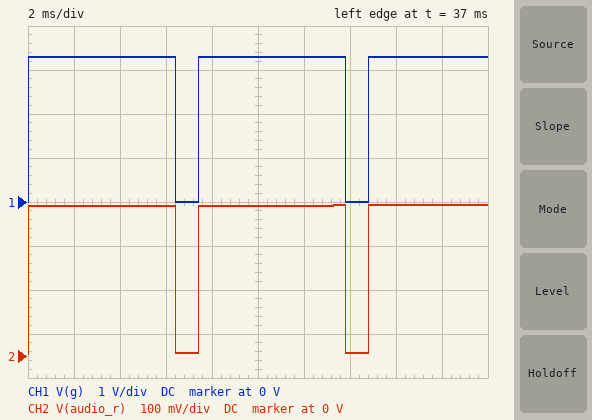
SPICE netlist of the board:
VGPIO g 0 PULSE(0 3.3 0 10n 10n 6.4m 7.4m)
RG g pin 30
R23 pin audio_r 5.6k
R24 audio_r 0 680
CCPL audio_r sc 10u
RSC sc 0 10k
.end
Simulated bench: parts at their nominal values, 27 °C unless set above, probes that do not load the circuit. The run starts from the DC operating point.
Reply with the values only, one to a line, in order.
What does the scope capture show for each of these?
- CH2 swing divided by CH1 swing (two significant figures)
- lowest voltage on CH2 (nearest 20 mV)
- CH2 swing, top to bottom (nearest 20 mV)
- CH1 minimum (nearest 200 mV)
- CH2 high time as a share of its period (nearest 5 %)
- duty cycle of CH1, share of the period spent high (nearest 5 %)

0.10
0 V
340 mV
0 V
85 %
85 %
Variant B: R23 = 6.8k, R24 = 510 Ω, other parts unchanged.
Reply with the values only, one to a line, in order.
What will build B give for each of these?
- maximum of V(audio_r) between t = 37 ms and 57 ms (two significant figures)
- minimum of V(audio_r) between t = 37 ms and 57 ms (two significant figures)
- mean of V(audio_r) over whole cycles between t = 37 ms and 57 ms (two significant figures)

220 mV
2.7 mV
190 mV
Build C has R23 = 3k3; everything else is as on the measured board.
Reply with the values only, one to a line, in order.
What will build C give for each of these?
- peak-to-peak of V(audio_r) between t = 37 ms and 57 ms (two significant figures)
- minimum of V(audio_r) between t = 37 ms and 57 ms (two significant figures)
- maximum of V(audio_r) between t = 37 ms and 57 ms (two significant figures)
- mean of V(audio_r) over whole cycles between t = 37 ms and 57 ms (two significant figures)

530 mV
7.6 mV
540 mV
470 mV
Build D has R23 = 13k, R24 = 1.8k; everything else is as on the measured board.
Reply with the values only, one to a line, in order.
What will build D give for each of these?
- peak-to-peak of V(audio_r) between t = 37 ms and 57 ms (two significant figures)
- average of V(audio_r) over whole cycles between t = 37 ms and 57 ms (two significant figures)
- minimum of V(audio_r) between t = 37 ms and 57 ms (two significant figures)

350 mV
310 mV
13 mV
